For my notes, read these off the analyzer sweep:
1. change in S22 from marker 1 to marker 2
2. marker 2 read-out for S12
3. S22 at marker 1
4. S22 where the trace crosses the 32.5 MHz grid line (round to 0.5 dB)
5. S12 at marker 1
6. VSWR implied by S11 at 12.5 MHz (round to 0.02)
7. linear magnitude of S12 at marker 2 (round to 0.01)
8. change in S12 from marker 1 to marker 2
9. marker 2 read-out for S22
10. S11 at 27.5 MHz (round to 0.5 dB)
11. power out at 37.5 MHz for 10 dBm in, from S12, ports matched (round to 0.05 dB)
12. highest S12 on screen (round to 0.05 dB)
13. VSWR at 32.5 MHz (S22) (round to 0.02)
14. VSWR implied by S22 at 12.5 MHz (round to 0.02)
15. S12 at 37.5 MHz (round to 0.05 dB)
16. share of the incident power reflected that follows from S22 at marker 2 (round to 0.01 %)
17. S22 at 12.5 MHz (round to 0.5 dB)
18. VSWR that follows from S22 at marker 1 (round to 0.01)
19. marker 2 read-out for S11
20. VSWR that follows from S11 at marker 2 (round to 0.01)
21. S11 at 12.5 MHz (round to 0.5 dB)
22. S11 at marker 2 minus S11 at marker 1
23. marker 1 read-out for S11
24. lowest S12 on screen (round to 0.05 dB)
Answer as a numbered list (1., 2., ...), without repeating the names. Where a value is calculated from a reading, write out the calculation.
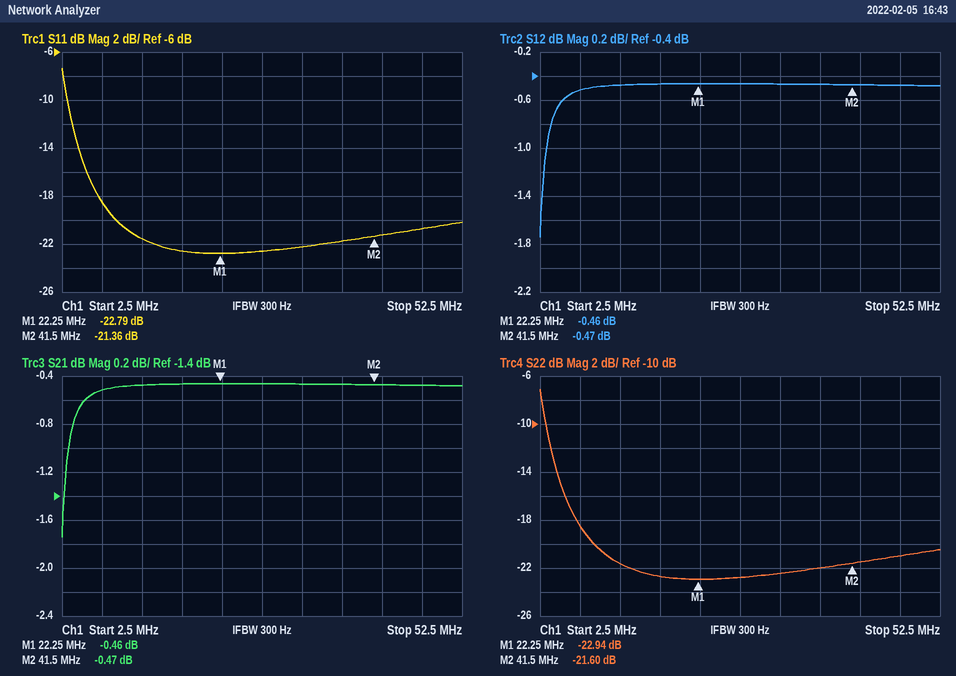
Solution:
1. -21.6 − (-22.94) = 1.34 dB
2. -0.47 dB
3. -22.94 dB
4. -22.5 dB
5. -0.46 dB
6. |Γ| = 10^(-21.5/20) = 0.0841; VSWR = (1 + 0.0841)/(1 − 0.0841) ≈ 1.18
7. 10^(-0.47/20) ≈ 0.95
8. -0.47 − (-0.46) = -0.01 dB
9. -21.60 dB
10. -22.5 dB
11. 10 dBm + (-0.45 dB) = 9.55 dBm
12. -0.45 dB
13. |Γ| = 10^(-22.5/20) = 0.0750; VSWR = (1 + 0.0750)/(1 − 0.0750) ≈ 1.16
14. |Γ| = 10^(-21.5/20) = 0.0841; VSWR = (1 + 0.0841)/(1 − 0.0841) ≈ 1.18
15. -0.45 dB
16. 10^(-21.6/10) ≈ 0.69 %
17. -21.5 dB
18. (1 + 0.0713)/(1 − 0.0713) ≈ 1.15
19. -21.36 dB
20. (1 + 0.0855)/(1 − 0.0855) ≈ 1.19
21. -21.5 dB
22. -21.36 − (-22.79) = 1.43 dB
23. -22.79 dB
24. -1.75 dB
